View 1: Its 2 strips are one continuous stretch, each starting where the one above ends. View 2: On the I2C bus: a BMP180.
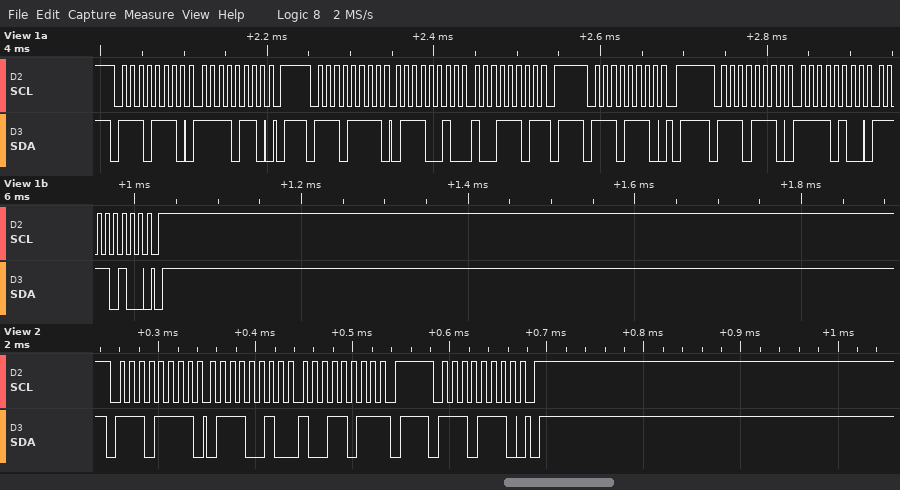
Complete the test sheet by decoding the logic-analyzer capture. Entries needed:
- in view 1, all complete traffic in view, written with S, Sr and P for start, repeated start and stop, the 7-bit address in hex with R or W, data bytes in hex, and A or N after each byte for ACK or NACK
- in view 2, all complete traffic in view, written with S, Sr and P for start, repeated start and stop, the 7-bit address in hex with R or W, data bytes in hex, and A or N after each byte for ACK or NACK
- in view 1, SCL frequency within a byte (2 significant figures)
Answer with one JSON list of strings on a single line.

["S 77W A F6 A P S 77R A 72 A 9D N P S 77W A P S 77W A F4 A F4 A P", "S 77R A 72 A 9B N P S 77W A P", "100 kHz"]
